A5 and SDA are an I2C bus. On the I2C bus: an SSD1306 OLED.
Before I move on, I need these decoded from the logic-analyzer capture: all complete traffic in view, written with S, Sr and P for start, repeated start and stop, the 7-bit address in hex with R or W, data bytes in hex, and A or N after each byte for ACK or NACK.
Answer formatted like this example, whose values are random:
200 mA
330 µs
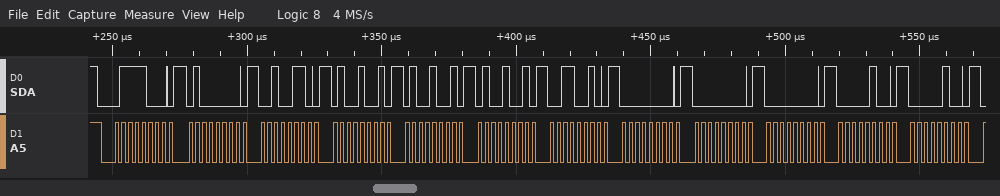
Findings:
S 3CW A 40 A 26 A 49 A 49 A 49 A 32 A 00 A 00 A 00 A 04 A 04 A
